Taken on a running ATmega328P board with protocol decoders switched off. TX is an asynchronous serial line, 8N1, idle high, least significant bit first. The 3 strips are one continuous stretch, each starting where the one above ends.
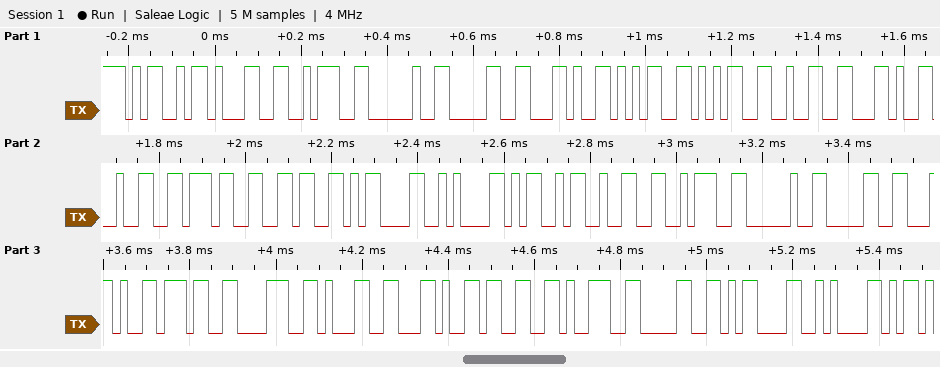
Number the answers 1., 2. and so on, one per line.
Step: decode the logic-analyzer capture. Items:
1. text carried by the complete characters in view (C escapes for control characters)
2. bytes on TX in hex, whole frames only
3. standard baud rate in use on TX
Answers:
1. "M1: 0,552,276\r\nM2: 0,781,390\r\n"
2. 4D 31 3A 20 30 2C 35 35 32 2C 32 37 36 0D 0A 4D 32 3A 20 30 2C 37 38 31 2C 33 39 30 0D 0A
3. 57600 baud
